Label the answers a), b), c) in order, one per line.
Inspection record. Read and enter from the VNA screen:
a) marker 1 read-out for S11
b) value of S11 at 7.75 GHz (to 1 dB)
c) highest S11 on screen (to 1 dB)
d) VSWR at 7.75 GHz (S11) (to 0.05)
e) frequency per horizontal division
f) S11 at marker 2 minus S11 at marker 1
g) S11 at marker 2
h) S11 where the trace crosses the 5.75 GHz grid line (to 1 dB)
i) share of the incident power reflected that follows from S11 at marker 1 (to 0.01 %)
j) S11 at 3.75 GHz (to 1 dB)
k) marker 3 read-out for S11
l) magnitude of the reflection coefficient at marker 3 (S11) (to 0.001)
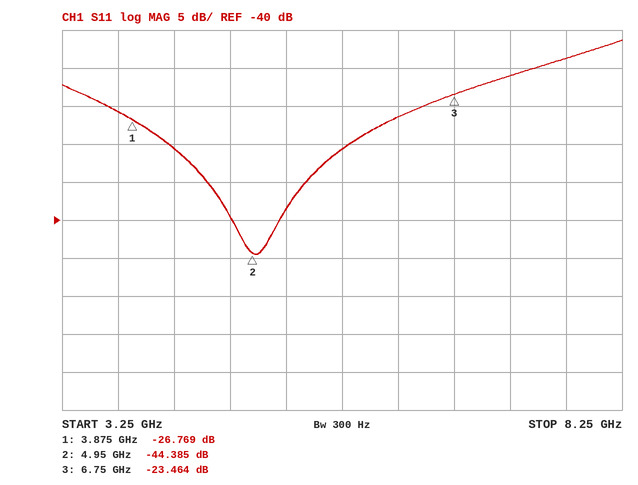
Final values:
a) -26.769 dB
b) -19 dB
c) -16 dB
d) 1.25
e) 500 MHz
f) -17.616 dB
g) -44.385 dB
h) -31 dB
i) 0.21 %
j) -26 dB
k) -23.464 dB
l) 0.067
